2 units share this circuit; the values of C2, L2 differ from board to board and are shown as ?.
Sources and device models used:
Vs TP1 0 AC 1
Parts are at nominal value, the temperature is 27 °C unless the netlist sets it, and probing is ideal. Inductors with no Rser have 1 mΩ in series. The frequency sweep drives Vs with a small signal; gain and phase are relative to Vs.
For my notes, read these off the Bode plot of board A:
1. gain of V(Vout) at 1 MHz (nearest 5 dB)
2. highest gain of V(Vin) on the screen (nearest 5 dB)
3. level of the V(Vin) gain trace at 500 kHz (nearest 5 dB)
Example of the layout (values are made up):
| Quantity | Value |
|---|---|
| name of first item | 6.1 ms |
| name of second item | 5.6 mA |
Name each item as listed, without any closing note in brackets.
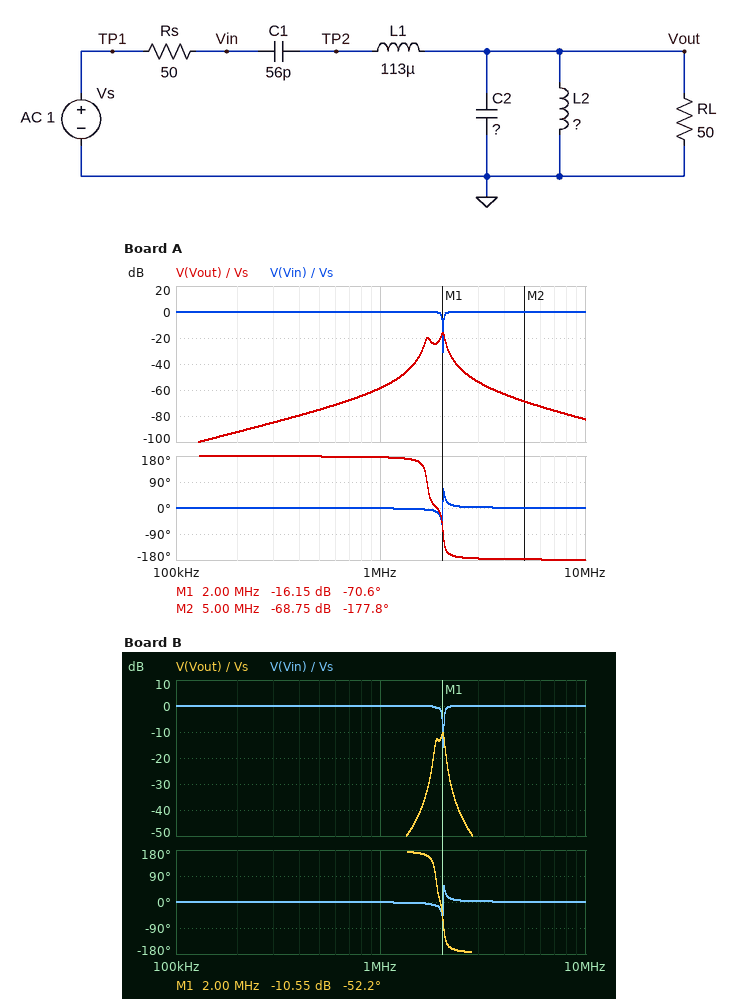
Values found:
| Quantity | Value |
|---|---|
| gain of V(Vout) at 1 MHz | -60 dB |
| highest gain of V(Vin) on the screen | 0 dB |
| level of the V(Vin) gain trace at 500 kHz | 0 dB |
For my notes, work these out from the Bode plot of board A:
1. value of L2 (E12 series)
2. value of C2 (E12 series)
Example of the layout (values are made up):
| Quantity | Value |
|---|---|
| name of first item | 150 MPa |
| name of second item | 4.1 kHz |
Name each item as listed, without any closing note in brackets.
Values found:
| Quantity | Value |
|---|---|
| value of L2 | 270 nH |
| value of C2 | 33 nF |
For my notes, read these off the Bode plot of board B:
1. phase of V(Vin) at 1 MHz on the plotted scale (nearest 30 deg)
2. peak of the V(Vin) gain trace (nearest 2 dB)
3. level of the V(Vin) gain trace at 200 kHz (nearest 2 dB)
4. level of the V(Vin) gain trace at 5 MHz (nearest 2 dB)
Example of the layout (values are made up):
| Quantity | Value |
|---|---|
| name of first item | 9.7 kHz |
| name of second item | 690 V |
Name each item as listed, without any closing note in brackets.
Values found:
| Quantity | Value |
|---|---|
| phase of V(Vin) at 1 MHz on the plotted scale | 0 deg |
| peak of the V(Vin) gain trace | 0 dB |
| level of the V(Vin) gain trace at 200 kHz | 0 dB |
| level of the V(Vin) gain trace at 5 MHz | 0 dB |
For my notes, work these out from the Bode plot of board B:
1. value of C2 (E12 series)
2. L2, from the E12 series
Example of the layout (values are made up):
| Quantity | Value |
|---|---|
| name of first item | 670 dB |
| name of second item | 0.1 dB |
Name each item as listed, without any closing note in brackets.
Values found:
| Quantity | Value |
|---|---|
| value of C2 | 33 nF |
| L2, from the E12 series | 220 nH |
